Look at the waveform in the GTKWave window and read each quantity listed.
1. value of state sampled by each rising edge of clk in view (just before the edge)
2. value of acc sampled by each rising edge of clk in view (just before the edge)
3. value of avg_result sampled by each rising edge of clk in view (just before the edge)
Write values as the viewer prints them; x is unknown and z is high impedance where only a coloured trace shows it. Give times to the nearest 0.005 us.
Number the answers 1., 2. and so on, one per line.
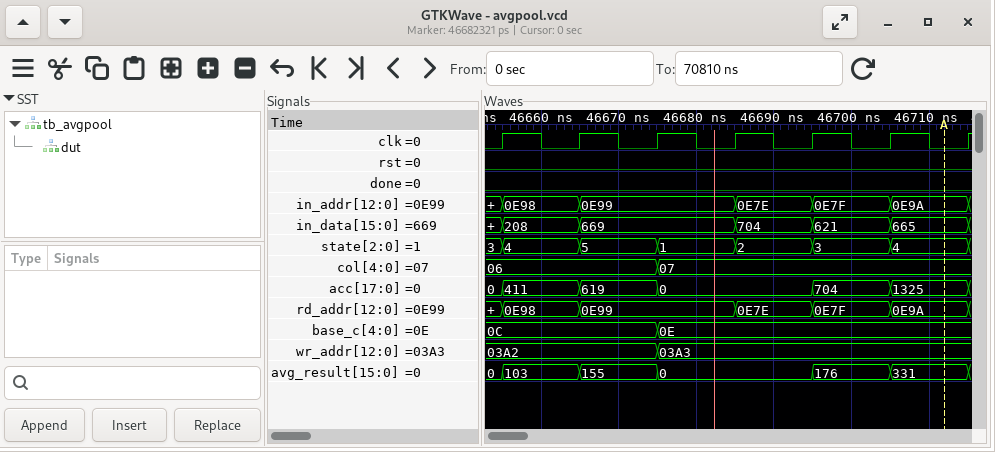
1. 3, 4, 5, 1, 2, 3, 4
2. 0, 411, 619, 0, 0, 704, 1325
3. 0, 103, 155, 0, 0, 176, 331
